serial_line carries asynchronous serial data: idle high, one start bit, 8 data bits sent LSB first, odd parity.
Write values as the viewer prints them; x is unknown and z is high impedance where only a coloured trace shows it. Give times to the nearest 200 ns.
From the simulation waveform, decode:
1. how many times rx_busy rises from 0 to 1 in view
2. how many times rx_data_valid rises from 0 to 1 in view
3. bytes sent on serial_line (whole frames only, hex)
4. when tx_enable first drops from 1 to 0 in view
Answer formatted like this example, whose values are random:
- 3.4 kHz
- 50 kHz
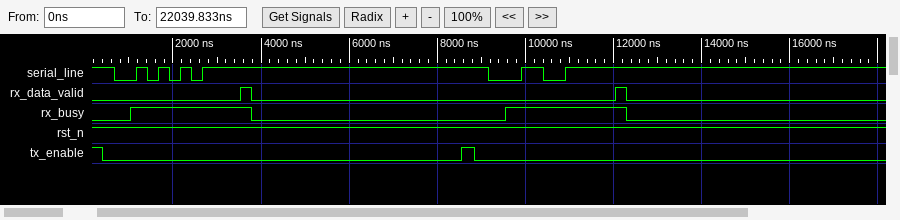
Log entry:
- 2
- 2
- AA, CC
- 400 ns
